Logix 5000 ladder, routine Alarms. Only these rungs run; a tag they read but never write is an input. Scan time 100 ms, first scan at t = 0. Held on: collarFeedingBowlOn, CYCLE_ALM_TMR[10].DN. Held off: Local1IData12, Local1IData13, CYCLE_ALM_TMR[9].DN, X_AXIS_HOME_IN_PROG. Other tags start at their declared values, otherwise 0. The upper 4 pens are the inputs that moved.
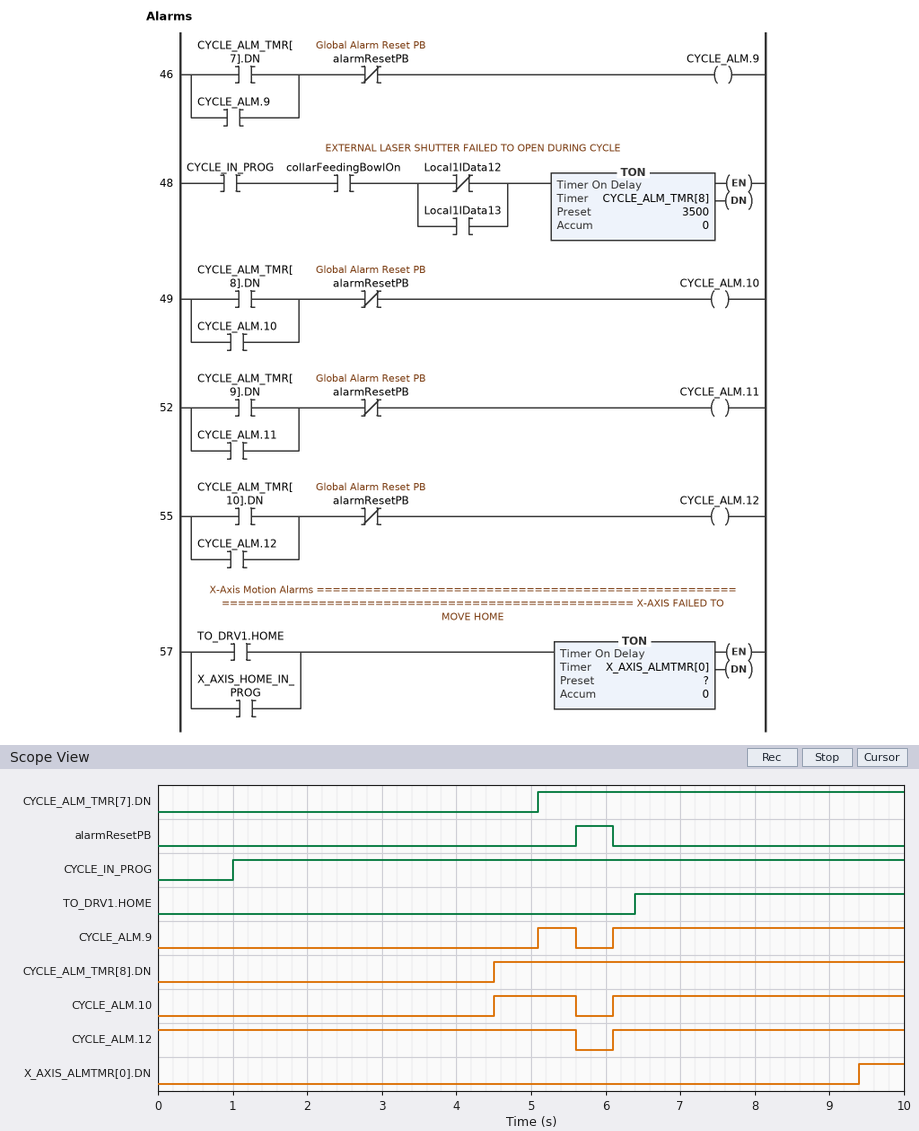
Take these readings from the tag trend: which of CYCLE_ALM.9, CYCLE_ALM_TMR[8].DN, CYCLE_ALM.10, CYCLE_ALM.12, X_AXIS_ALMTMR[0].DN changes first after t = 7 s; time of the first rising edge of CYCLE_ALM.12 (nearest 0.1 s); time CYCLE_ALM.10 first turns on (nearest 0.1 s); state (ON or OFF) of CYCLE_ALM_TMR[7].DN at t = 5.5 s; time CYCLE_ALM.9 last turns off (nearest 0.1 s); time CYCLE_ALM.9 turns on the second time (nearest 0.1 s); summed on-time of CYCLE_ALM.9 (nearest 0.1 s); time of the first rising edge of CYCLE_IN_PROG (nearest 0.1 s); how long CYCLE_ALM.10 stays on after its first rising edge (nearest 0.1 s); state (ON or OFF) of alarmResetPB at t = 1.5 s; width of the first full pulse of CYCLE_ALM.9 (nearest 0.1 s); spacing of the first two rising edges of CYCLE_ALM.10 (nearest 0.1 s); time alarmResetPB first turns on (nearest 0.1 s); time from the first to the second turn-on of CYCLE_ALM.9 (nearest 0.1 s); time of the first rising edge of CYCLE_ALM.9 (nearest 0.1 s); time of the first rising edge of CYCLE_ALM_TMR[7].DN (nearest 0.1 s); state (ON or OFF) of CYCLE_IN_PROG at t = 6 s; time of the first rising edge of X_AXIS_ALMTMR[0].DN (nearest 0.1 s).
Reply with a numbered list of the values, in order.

1. X_AXIS_ALMTMR[0].DN
2. 6.1 s
3. 4.5 s
4. ON
5. 5.6 s
6. 6.1 s
7. 4.4 s
8. 1.0 s
9. 1.1 s
10. OFF
11. 0.5 s
12. 1.6 s
13. 5.6 s
14. 1.0 s
15. 5.1 s
16. 5.1 s
17. ON
18. 9.4 s
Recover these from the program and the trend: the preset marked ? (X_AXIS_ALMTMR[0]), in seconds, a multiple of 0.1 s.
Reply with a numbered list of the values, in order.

1. 3.0 s
